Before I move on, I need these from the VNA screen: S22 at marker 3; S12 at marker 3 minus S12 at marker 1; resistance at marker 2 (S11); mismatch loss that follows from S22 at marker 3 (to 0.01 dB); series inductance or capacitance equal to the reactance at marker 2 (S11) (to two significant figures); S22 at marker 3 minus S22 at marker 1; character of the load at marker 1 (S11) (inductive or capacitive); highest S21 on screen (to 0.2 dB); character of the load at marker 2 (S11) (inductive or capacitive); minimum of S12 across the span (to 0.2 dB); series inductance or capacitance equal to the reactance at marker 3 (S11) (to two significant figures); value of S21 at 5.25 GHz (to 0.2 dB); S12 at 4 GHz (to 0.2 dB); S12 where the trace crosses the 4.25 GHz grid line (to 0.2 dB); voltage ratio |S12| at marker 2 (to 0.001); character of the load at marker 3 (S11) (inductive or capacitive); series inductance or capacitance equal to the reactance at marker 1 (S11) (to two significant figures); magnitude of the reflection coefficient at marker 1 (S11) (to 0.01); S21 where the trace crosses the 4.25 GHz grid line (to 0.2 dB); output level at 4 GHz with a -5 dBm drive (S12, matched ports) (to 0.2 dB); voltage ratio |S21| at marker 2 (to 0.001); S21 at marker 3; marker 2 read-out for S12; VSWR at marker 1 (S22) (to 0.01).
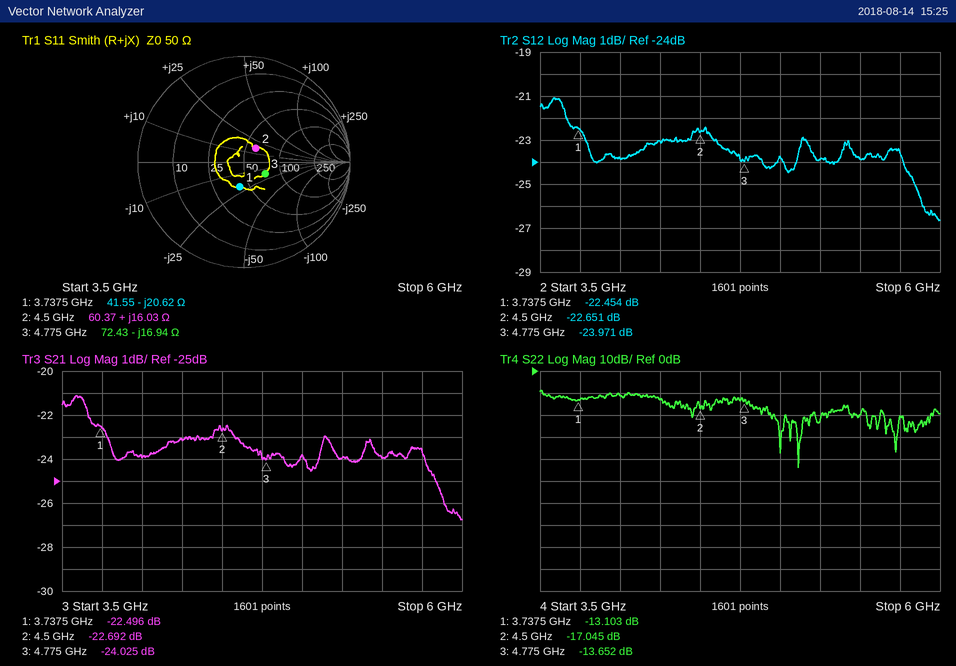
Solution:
-13.652 dB
-1.517 dB
60.37 Ω
0.19 dB
570 pH
-0.549 dB
capacitive
-21.2 dB
inductive
-26.6 dB
2.0 pF
-24.0 dB
-23.8 dB
-23.0 dB
0.074
capacitive
2.1 pF
0.24
-23.2 dB
-28.8 dBm
0.073
-24.025 dB
-22.651 dB
1.57
